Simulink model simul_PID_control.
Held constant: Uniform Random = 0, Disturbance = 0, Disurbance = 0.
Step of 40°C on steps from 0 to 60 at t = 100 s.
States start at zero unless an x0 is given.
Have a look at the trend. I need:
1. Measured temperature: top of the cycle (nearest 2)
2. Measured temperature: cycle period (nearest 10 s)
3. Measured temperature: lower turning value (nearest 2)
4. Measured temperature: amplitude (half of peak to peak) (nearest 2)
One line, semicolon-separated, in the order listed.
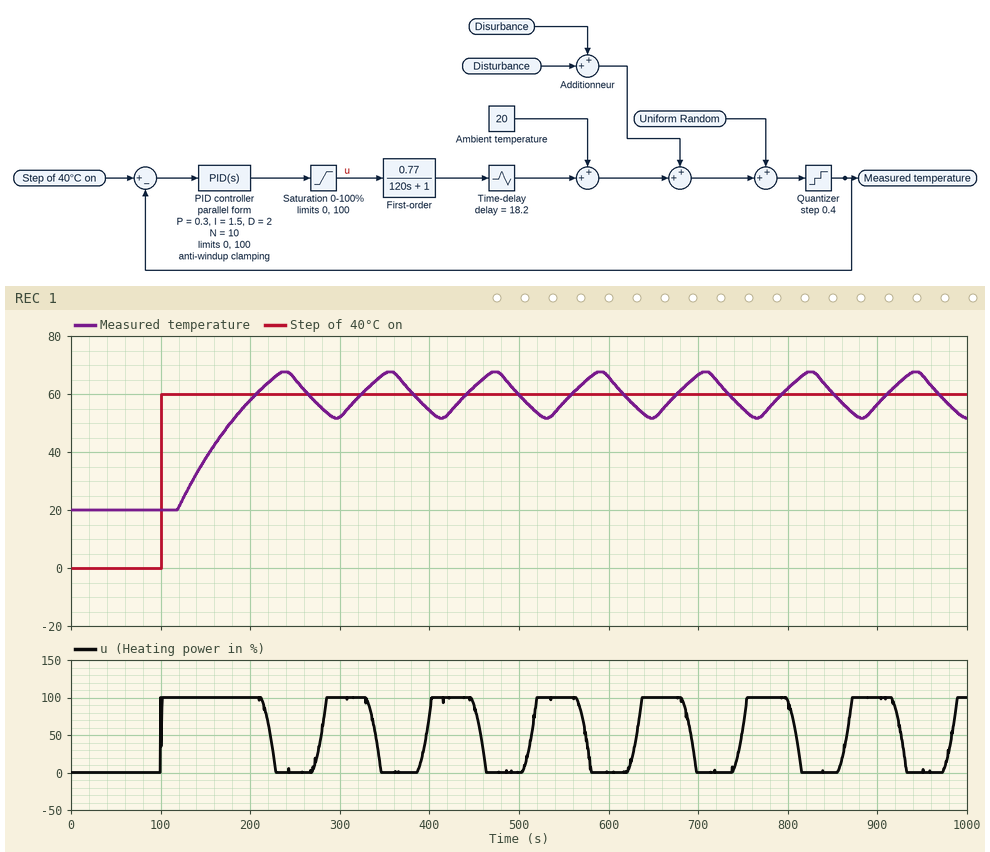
68; 120 s; 52; 8
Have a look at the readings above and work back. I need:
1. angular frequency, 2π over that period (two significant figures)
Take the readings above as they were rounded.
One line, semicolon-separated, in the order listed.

0.052 rad/s
